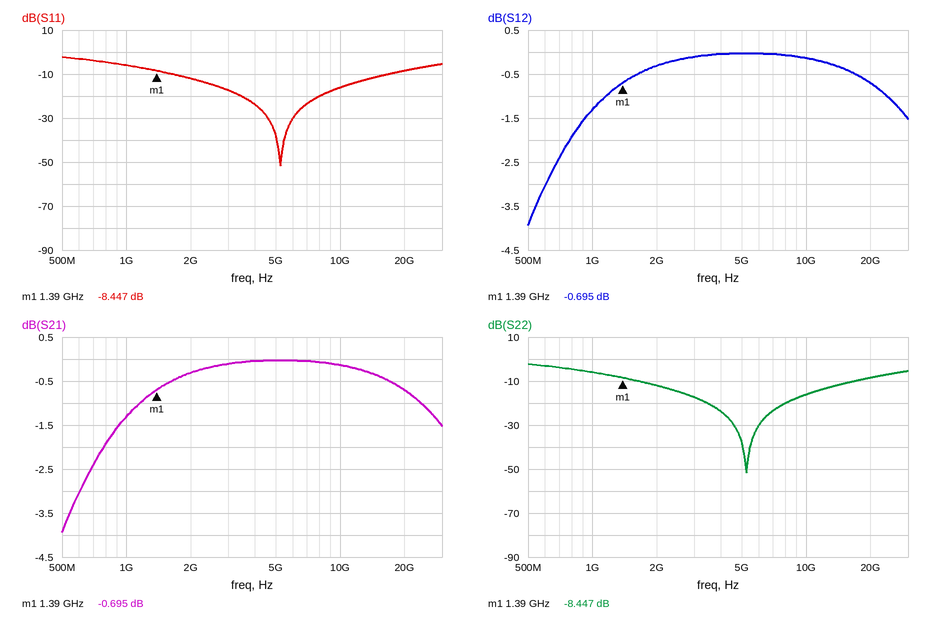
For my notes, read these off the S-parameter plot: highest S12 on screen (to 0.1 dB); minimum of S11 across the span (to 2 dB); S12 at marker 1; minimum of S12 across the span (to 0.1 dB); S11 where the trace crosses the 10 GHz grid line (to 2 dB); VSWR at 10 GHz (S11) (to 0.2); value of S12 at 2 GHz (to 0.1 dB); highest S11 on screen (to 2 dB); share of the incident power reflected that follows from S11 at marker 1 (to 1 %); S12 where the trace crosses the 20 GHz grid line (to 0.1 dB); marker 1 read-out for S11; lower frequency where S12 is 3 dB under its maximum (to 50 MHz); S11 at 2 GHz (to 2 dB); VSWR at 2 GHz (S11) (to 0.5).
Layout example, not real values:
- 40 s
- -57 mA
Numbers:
- 0.0 dB
- -52 dB
- -0.695 dB
- -3.9 dB
- -16 dB
- 1.4
- -0.3 dB
- -2 dB
- 14 %
- -0.7 dB
- -8.447 dB
- 600 MHz
- -12 dB
- 1.5
